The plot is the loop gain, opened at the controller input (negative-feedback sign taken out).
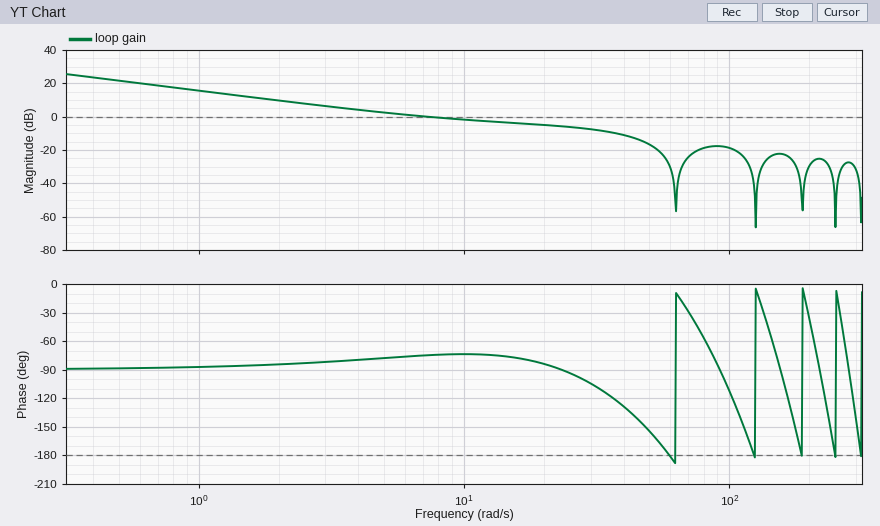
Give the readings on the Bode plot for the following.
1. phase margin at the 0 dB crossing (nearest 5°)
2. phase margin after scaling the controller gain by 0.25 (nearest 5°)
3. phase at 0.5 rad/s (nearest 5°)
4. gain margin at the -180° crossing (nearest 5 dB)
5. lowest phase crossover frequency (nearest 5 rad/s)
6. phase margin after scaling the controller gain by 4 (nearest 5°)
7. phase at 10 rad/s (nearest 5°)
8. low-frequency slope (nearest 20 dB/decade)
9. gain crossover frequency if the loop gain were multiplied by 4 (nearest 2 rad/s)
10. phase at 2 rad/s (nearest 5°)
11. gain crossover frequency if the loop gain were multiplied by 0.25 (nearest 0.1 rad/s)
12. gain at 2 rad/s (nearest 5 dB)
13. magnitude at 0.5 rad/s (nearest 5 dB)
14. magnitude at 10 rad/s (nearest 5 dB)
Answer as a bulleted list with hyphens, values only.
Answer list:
- 105°
- 95°
- -90°
- 30 dB
- 60 rad/s
- 45°
- -75°
- -20 dB/decade
- 42 rad/s
- -85°
- 1.5 rad/s
- 10 dB
- 20 dB
- 0 dB
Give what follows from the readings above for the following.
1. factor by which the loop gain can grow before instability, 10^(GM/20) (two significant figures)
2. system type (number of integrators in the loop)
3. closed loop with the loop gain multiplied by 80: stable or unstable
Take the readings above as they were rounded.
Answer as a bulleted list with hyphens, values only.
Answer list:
- 32
- 1
- unstable
